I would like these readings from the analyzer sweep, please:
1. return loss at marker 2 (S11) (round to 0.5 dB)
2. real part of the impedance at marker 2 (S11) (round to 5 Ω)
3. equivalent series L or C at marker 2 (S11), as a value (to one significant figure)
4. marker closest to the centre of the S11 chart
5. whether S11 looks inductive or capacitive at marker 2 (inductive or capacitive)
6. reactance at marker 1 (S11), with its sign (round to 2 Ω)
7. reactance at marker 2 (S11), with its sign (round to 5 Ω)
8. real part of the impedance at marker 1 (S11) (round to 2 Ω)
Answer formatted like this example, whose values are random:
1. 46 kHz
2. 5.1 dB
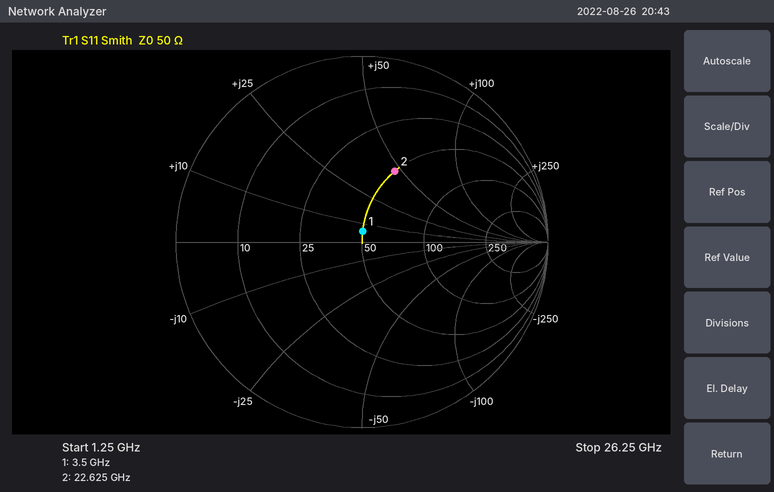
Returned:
1. 7.5 dB
2. 50 Ω
3. 300 pH
4. marker 1
5. inductive
6. +6 Ω
7. +45 Ω
8. 50 Ω
